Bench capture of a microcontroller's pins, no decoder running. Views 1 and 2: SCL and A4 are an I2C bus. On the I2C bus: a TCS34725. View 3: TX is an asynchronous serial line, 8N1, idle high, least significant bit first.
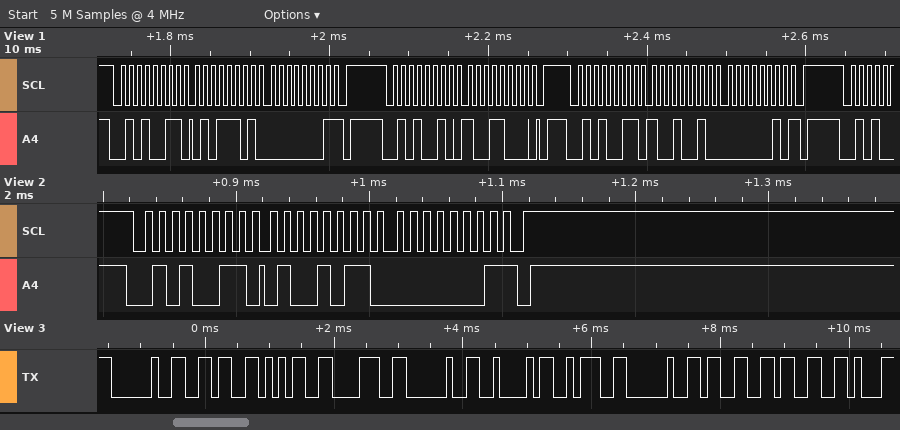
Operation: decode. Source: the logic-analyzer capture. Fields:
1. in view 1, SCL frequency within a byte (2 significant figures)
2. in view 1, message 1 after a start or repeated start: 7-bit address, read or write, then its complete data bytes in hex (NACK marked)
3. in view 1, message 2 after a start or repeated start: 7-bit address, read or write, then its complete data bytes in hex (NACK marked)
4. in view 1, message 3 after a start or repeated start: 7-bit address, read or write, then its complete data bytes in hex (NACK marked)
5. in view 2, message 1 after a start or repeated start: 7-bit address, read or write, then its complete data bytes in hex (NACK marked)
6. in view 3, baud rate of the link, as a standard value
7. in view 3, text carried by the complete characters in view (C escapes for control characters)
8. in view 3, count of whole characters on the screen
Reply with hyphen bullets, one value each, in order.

- 100 kHz
- 0x29 read: 5D 01 NACK
- 0x29 write: 98
- 0x29 read: 92 02 NACK
- 0x29 read: 4B 01 NACK
- 9600 baud
- " 658 B: 33"
- 10
